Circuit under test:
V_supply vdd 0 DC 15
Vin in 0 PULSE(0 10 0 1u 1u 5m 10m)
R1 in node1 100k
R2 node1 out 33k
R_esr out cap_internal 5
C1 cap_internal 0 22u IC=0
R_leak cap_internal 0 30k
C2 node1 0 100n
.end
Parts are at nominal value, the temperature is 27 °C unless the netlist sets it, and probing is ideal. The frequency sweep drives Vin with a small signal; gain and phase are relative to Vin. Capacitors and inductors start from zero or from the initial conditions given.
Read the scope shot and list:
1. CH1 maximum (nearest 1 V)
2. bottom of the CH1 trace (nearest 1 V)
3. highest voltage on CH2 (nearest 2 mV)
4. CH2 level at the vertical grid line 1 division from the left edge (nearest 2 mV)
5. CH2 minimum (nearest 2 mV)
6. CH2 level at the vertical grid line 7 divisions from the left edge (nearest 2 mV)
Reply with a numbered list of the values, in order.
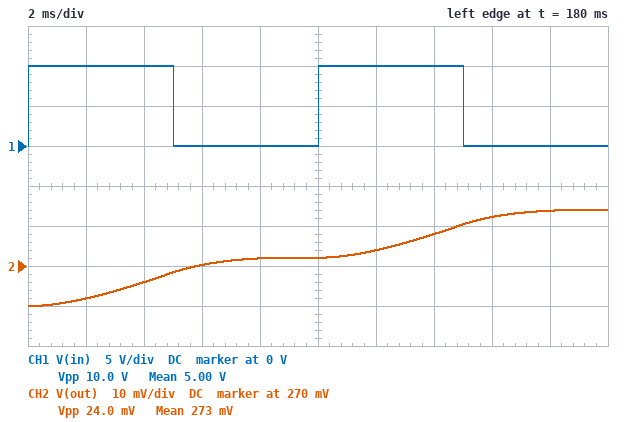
1. 10 V
2. 0 V
3. 284 mV
4. 262 mV
5. 260 mV
6. 278 mV
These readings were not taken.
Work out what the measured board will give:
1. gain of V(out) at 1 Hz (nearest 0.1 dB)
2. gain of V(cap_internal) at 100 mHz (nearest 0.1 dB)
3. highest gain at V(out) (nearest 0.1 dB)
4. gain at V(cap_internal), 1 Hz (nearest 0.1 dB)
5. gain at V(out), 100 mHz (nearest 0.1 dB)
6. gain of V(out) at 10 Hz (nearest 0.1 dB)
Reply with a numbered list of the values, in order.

1. -25.7 dB
2. -15.2 dB
3. -14.7 dB
4. -25.7 dB
5. -15.2 dB
6. -45.4 dB
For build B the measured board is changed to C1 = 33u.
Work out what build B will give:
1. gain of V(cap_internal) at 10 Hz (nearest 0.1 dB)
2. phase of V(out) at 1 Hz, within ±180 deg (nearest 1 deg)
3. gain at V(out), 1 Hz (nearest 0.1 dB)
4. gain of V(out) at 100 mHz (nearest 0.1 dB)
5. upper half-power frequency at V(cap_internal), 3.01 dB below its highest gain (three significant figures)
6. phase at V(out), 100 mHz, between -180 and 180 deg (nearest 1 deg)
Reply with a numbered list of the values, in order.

1. -48.9 dB
2. -80 deg
3. -29.0 dB
4. -15.7 dB
5. 197 mHz
6. -27 deg
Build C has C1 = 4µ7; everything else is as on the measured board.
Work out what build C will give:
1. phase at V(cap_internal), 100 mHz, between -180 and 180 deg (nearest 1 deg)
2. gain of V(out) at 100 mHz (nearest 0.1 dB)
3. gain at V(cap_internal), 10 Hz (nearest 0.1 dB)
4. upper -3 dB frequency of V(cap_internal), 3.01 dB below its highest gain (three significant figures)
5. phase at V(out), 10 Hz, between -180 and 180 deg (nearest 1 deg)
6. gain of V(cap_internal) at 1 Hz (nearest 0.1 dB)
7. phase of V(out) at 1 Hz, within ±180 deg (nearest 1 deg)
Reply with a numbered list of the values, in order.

1. -4 deg
2. -14.7 dB
3. -32.2 dB
4. 1.37 Hz
5. -91 deg
6. -16.6 dB
7. -37 deg
